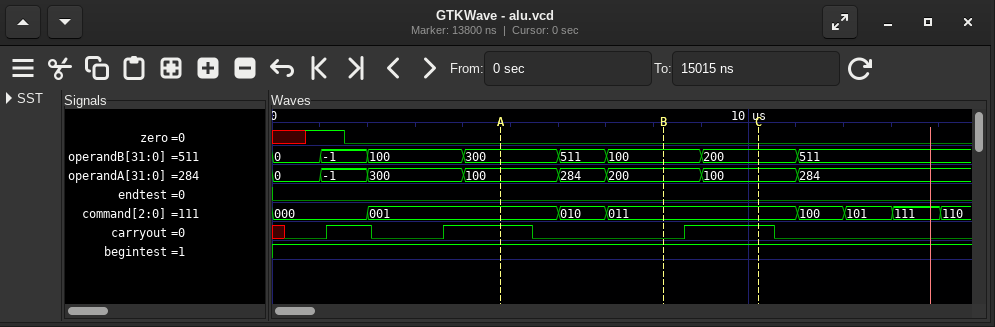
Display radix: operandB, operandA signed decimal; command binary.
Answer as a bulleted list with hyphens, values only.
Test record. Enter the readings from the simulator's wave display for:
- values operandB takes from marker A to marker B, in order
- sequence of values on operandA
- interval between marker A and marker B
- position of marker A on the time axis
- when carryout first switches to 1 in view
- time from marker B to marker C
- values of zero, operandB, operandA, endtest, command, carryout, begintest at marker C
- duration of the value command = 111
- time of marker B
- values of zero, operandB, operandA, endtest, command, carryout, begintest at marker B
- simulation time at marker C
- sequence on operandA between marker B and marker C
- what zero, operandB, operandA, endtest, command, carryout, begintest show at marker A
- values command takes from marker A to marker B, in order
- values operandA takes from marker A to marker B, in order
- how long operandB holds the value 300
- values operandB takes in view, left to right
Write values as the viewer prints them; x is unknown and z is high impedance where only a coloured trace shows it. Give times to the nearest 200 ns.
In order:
- 300, 511, 100
- 0, -1, 300, 100, 284, 200, 100, 284
- 3400 ns
- 4800 ns
- 1200 ns
- 2000 ns
- zero=0, operandB=200, operandA=100, endtest=0, command=011, carryout=1, begintest=1
- 1000 ns
- 8200 ns
- zero=0, operandB=100, operandA=200, endtest=0, command=011, carryout=0, begintest=1
- 10200 ns
- 200, 100
- zero=0, operandB=300, operandA=100, endtest=0, command=001, carryout=1, begintest=1
- 001, 010, 011
- 100, 284, 200
- 2000 ns
- 0, -1, 100, 300, 511, 100, 200, 511
